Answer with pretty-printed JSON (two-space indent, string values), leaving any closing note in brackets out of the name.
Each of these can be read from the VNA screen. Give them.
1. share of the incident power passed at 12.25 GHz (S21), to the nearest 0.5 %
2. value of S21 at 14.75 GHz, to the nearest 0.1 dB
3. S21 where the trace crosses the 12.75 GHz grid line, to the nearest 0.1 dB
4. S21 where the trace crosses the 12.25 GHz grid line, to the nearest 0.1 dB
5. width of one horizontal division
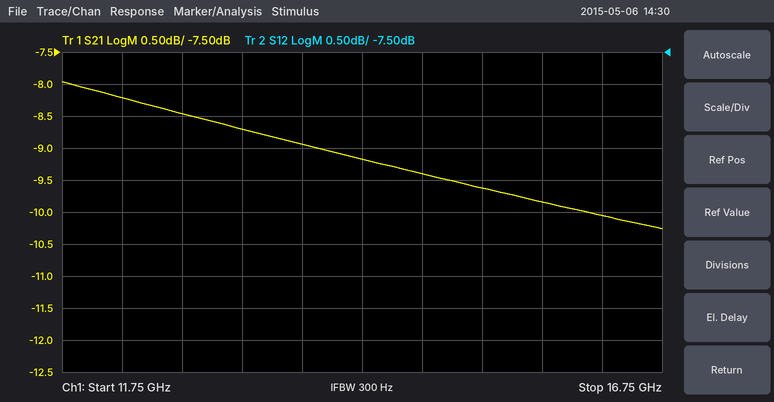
{
  "share of the incident power passed at 12.25 GHz (S21), to the nearest 0.5 %": "15.0 %",
  "value of S21 at 14.75 GHz, to the nearest 0.1 dB": "-9.4 dB",
  "S21 where the trace crosses the 12.75 GHz grid line, to the nearest 0.1 dB": "-8.5 dB",
  "S21 where the trace crosses the 12.25 GHz grid line, to the nearest 0.1 dB": "-8.2 dB",
  "width of one horizontal division": "500 MHz"
}
